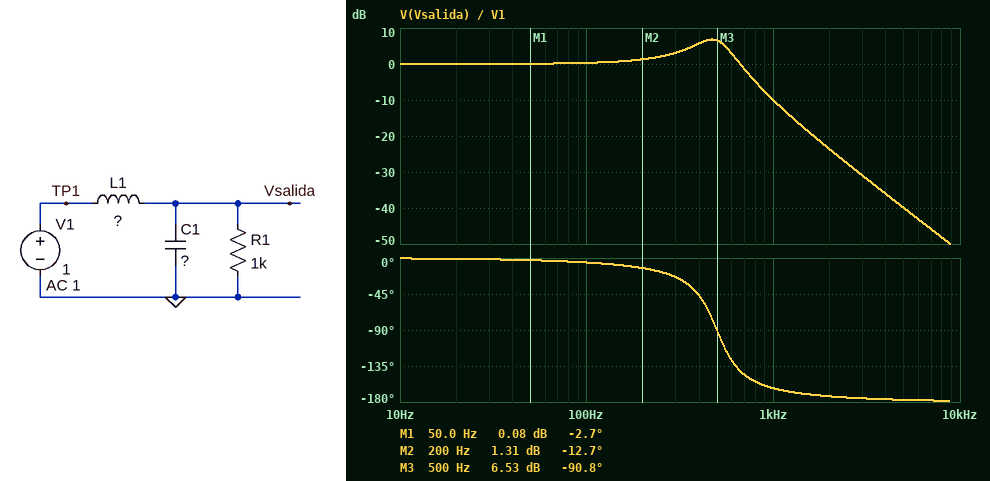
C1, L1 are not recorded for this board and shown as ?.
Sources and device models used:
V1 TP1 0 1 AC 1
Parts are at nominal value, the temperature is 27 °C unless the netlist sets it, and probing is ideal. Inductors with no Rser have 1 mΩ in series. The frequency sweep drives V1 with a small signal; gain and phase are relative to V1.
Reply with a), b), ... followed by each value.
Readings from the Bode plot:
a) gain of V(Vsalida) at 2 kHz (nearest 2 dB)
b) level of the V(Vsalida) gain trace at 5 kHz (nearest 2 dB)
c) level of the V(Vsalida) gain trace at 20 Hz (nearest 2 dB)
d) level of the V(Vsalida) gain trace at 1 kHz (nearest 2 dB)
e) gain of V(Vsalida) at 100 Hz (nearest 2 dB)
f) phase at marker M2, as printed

a) -24 dB
b) -40 dB
c) 0 dB
d) -10 dB
e) 0 dB
f) -12.7 deg
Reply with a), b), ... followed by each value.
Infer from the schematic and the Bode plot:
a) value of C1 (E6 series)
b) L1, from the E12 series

a) 680 nF
b) 150 mH
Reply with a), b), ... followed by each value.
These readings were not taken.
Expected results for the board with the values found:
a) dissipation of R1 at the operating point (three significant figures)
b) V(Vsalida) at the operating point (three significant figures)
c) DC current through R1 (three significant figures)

a) 1.00 mW
b) 1.00 V
c) 1.00 mA
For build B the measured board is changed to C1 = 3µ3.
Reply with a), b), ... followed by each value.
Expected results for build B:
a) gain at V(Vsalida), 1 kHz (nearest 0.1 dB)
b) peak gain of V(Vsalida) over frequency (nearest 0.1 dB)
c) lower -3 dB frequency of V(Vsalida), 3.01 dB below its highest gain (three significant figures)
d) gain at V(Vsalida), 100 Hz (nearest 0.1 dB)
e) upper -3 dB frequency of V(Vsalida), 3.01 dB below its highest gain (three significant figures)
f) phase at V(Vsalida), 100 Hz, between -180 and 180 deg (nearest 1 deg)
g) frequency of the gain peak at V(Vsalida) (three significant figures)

a) -25.4 dB
b) 13.5 dB
c) 198 Hz
d) 1.8 dB
e) 247 Hz
f) -7 deg
g) 224 Hz
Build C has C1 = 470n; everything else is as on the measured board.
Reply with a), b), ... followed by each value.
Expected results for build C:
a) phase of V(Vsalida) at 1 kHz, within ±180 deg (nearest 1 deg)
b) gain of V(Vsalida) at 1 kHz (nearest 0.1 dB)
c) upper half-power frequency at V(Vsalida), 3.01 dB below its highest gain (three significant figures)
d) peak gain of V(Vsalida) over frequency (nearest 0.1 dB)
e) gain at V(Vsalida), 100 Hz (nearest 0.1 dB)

a) -152 deg
b) -6.1 dB
c) 705 Hz
d) 5.3 dB
e) 0.2 dB
